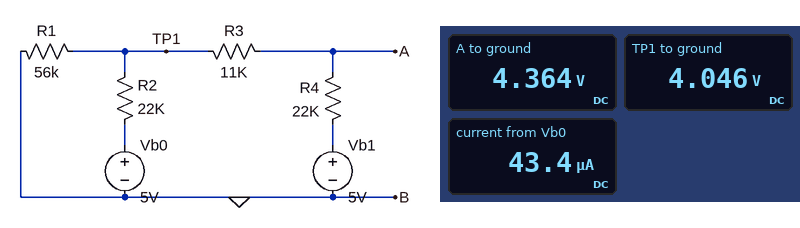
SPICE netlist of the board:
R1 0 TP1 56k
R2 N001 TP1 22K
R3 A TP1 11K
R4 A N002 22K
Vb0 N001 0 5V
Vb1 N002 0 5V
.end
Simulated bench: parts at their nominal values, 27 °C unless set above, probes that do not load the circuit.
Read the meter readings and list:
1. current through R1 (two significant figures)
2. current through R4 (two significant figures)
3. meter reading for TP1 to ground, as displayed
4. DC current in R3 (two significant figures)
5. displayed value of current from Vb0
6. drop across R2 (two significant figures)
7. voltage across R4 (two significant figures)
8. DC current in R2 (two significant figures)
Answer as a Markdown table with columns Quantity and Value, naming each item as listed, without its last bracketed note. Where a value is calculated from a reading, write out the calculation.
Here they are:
| Quantity | Value |
|---|---|
| current through R1 | (4.046 V) / 56 kΩ = 72 µA |
| current through R4 | (5 V - 4.364 V) / 22 kΩ = 29 µA |
| meter reading for TP1 to ground, as displayed | 4.046 V |
| DC current in R3 | (4.364 V - 4.046 V) / 11 kΩ = 29 µA |
| displayed value of current from Vb0 | 43.4 µA |
| drop across R2 | 5 V - 4.046 V = 950 mV |
| voltage across R4 | 5 V - 4.364 V = 640 mV |
| DC current in R2 | (5 V - 4.046 V) / 22 kΩ = 43 µA |
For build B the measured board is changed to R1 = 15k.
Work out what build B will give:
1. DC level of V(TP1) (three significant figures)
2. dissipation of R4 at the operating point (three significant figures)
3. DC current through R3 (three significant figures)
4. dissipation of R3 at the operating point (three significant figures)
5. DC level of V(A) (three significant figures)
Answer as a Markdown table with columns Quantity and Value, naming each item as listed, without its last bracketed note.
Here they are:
| Quantity | Value |
|---|---|
| DC level of V(TP1) | 2.66 V |
| dissipation of R4 at the operating point | 111 µW |
| DC current through R3 | 70.9 µA |
| dissipation of R3 at the operating point | 55.3 µW |
| DC level of V(A) | 3.44 V |
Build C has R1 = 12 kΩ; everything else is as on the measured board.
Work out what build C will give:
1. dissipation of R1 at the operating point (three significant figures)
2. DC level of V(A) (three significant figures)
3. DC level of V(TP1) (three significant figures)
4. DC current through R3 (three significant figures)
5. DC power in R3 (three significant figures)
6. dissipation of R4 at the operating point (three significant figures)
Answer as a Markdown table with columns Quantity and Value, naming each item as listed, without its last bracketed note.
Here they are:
| Quantity | Value |
|---|---|
| dissipation of R1 at the operating point | 472 µW |
| DC level of V(A) | 3.25 V |
| DC level of V(TP1) | 2.38 V |
| DC current through R3 | 79.4 µA |
| DC power in R3 | 69.3 µW |
| dissipation of R4 at the operating point | 139 µW |
